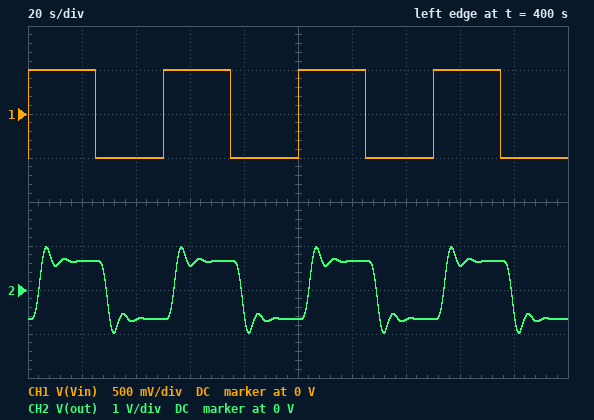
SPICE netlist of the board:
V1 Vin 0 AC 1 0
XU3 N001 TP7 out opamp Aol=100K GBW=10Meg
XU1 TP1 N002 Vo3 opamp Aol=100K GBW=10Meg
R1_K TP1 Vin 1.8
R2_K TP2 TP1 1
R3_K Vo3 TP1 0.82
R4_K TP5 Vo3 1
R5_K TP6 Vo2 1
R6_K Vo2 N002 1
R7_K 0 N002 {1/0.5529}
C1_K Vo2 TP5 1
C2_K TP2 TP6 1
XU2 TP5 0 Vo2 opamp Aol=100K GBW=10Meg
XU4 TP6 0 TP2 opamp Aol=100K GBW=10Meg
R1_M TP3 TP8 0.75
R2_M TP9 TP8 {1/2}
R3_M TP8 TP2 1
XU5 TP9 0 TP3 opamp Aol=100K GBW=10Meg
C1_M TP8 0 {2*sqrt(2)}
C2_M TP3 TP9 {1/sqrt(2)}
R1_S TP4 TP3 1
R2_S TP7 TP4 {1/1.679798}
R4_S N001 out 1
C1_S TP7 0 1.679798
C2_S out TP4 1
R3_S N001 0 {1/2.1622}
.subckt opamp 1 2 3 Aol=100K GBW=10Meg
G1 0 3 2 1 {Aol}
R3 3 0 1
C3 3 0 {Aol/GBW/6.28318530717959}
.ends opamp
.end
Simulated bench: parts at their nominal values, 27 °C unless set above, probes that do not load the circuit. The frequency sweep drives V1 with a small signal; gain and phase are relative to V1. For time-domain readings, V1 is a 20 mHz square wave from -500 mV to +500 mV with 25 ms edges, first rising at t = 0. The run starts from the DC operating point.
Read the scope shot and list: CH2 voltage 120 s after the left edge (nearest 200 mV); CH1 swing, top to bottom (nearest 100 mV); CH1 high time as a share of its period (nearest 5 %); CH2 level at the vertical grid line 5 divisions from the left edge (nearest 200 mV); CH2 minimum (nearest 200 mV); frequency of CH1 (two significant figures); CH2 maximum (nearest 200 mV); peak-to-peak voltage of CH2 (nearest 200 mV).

600 mV
1.0 V
50 %
-600 mV
-1.0 V
20 mHz
1.0 V
2.0 V
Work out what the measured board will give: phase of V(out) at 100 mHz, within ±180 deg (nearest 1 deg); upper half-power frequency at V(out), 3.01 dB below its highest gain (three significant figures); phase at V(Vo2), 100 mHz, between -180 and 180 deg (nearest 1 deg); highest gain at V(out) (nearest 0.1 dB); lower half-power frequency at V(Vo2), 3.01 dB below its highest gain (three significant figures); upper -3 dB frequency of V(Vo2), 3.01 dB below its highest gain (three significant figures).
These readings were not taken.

-139 deg
163 mHz
25 deg
4.0 dB
68.8 mHz
302 mHz
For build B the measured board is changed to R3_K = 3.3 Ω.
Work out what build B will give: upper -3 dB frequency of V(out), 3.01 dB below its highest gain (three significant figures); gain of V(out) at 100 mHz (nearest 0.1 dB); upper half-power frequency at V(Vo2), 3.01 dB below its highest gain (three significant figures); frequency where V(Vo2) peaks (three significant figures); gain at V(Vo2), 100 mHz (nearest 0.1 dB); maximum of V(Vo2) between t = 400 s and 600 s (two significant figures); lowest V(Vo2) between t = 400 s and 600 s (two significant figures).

170 mHz
4.3 dB
741 mHz
289 mHz
-10.4 dB
350 mV
-350 mV
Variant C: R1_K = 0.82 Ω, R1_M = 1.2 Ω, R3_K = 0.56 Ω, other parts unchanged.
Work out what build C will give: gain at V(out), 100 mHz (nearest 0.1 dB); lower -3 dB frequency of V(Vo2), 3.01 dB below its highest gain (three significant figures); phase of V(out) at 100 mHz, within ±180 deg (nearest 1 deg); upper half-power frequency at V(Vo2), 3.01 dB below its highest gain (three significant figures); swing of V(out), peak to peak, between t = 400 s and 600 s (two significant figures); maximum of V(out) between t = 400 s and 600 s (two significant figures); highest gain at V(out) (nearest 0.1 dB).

11.0 dB
50.6 mHz
-171 deg
280 mHz
5.0 V
2.5 V
13.3 dB
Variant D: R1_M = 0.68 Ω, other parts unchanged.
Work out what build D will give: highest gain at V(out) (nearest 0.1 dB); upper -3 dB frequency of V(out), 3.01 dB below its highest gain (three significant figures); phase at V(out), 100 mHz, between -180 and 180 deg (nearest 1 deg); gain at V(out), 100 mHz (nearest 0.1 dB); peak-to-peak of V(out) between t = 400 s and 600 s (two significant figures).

3.3 dB
164 mHz
-136 deg
3.0 dB
1.8 V
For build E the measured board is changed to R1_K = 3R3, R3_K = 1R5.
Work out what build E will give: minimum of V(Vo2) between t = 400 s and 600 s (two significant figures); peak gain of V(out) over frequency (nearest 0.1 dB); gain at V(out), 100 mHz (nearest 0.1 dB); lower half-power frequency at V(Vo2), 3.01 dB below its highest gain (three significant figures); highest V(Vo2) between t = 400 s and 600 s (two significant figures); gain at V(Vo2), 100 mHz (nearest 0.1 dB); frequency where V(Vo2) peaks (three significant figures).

-160 mV
0.6 dB
-0.4 dB
95.4 mHz
160 mV
-15.1 dB
195 mHz
